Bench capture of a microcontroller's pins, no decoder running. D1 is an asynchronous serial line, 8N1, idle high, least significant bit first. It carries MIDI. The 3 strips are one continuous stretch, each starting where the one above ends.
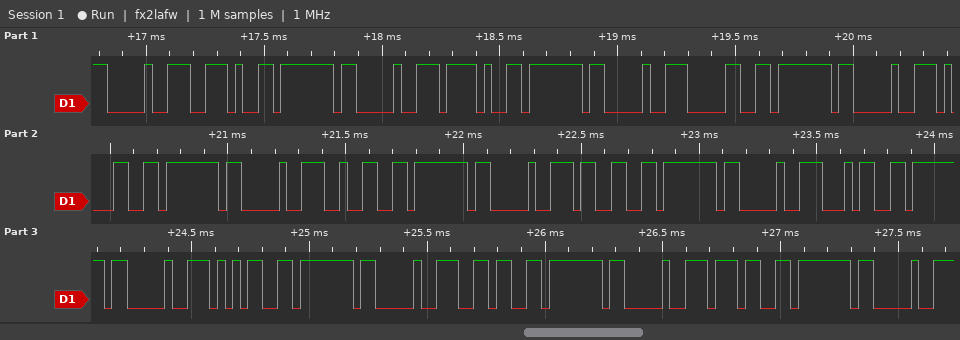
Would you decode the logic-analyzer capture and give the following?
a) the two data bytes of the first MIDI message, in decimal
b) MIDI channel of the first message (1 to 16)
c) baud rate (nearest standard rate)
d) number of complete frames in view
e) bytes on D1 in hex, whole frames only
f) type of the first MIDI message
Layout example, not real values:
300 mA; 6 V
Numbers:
46, 127; 1; 31250 baud; 31; 90 2E 7F 90 2F 7F 90 30 7F 90 31 7F 90 32 7F 90 33 7F 90 34 7F 90 35 7F 90 36 7F 90 37 7F 90; Note On
